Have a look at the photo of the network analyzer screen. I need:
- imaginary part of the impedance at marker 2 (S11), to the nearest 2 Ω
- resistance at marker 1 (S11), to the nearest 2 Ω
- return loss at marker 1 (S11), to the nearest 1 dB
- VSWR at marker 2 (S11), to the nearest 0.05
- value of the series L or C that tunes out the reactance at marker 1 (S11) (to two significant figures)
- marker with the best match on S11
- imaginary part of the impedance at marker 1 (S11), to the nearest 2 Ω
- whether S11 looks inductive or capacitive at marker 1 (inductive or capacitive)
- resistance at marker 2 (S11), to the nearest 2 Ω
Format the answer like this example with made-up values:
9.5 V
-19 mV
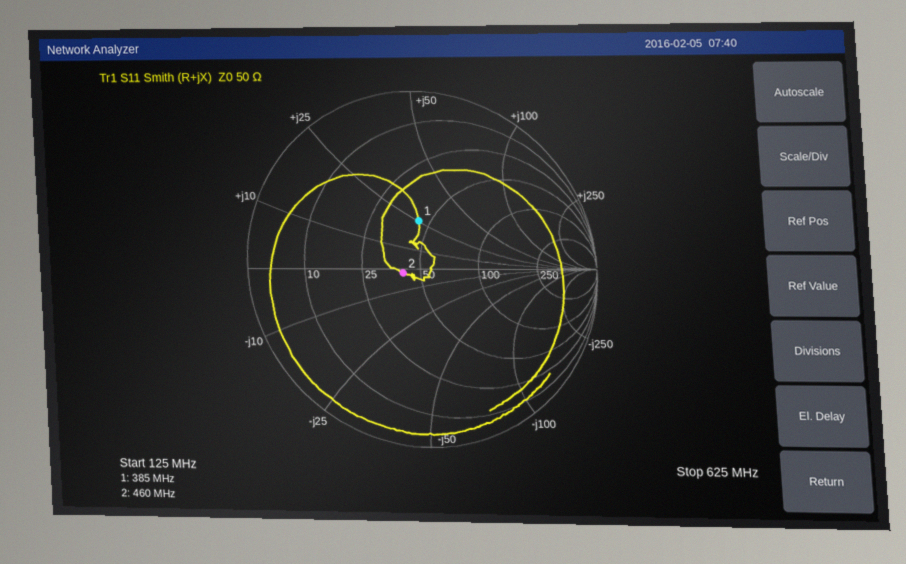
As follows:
-2 Ω
44 Ω
11 dB
1.25
16 pF
marker 2
+26 Ω
inductive
40 Ω
